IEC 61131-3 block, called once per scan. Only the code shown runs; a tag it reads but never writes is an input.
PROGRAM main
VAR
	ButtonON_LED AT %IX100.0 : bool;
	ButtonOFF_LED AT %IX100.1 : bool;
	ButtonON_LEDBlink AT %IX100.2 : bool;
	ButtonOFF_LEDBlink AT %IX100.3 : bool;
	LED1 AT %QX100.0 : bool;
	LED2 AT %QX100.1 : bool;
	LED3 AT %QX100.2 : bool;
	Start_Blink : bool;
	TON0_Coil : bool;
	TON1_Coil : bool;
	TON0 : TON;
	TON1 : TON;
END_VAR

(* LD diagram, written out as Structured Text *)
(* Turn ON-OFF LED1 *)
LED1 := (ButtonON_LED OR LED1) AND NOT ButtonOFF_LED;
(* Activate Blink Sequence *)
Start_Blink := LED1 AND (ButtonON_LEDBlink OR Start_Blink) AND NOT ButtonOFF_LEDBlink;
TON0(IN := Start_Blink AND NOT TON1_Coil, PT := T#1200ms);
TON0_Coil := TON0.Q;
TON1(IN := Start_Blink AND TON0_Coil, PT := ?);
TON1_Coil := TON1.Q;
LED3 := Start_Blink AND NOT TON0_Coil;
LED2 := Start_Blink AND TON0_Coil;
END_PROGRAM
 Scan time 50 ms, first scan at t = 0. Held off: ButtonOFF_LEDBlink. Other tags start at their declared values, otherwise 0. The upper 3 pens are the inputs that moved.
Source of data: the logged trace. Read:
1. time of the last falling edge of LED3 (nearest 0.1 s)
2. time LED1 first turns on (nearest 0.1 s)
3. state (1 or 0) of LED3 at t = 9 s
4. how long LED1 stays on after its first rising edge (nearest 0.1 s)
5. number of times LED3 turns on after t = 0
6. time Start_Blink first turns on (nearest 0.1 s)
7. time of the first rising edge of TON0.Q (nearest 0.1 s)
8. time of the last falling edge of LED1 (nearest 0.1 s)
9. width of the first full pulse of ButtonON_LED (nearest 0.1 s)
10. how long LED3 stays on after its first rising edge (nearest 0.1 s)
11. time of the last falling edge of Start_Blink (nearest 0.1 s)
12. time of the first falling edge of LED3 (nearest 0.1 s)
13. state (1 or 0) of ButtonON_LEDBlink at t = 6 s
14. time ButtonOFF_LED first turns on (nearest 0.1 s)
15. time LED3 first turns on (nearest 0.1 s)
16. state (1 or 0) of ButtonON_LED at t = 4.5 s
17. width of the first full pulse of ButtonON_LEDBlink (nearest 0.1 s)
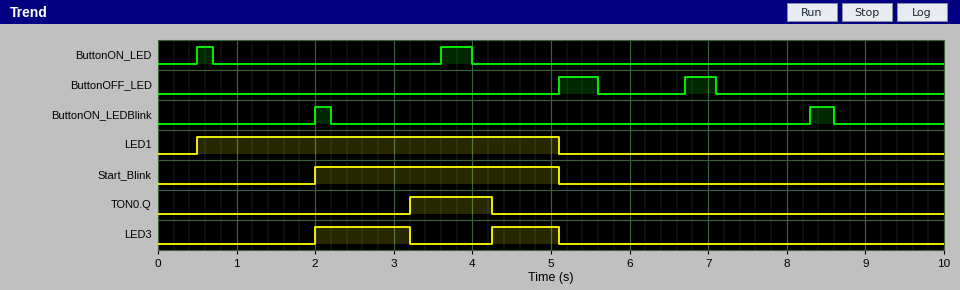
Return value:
5.1 s
0.5 s
0
4.6 s
2
2.0 s
3.2 s
5.1 s
0.2 s
1.2 s
5.1 s
3.2 s
0
5.1 s
2.0 s
0
0.2 s
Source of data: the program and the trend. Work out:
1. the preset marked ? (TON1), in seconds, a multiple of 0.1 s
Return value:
1.0 s
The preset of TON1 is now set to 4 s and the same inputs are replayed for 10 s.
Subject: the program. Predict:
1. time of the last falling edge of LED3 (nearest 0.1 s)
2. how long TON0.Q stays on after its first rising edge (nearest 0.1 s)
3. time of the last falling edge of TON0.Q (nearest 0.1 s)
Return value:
3.2 s
1.9 s
5.1 s
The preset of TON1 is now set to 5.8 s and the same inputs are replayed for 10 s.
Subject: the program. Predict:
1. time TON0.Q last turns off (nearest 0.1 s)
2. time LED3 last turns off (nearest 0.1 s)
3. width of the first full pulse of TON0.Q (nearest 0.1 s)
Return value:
5.1 s
3.2 s
1.9 s
